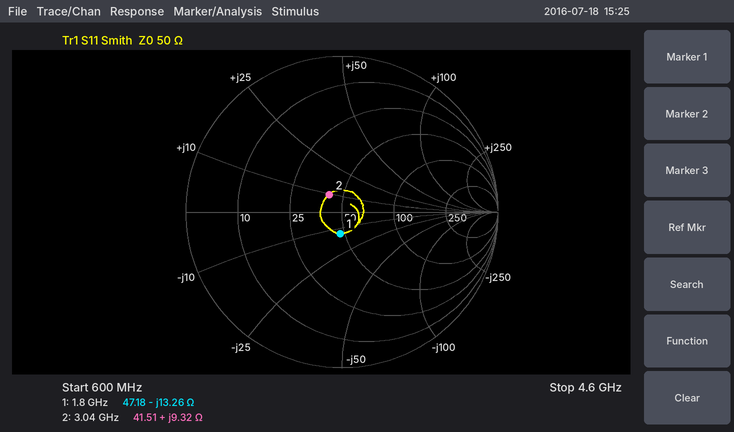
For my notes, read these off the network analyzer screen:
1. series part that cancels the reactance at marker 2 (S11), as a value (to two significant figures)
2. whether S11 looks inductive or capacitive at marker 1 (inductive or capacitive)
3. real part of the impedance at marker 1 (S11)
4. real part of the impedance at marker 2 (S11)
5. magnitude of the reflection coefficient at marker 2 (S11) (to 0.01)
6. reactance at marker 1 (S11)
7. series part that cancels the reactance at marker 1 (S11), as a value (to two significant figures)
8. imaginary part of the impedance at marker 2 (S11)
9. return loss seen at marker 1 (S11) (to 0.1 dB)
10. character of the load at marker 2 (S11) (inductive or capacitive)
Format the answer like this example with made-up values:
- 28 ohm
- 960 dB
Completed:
- 5.6 pF
- capacitive
- 47.18 Ω
- 41.51 Ω
- 0.14
- -13.26 Ω
- 1.2 nH
- +9.32 Ω
- 17.2 dB
- inductive
